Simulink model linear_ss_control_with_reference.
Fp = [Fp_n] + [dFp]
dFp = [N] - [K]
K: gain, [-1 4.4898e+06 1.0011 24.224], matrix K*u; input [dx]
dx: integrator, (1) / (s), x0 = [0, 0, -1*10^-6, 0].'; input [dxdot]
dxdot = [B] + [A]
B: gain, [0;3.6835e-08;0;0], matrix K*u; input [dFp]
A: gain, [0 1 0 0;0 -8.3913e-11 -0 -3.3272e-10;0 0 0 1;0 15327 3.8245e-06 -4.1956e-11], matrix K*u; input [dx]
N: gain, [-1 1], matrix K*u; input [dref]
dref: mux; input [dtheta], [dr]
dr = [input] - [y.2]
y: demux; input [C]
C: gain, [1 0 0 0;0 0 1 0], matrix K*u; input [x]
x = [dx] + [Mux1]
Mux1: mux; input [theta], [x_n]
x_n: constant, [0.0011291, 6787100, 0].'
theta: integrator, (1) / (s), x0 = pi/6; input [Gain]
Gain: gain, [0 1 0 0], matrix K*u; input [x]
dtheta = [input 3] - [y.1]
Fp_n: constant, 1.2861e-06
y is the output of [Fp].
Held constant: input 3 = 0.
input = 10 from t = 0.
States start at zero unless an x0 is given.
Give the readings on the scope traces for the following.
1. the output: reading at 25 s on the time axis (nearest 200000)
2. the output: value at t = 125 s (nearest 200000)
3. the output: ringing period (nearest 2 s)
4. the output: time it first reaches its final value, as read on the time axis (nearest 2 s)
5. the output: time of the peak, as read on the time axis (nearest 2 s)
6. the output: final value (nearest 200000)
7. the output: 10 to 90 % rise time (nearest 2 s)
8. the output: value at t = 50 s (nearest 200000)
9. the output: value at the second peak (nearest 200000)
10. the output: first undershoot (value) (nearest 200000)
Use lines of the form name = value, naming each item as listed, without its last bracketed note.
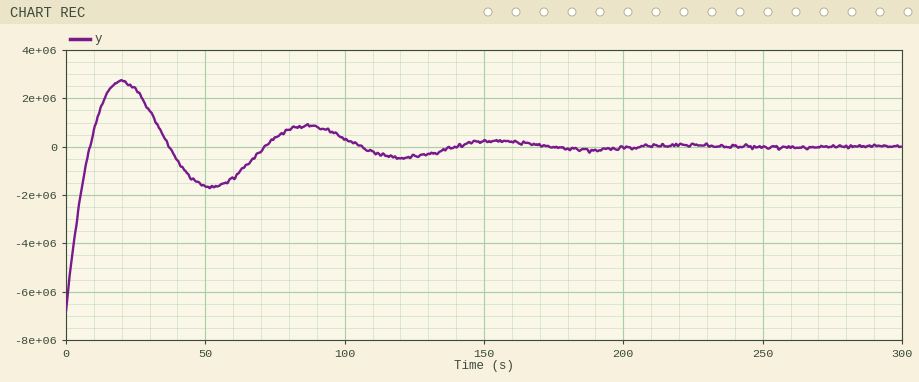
the output: reading at 25 s on the time axis = 2400000
the output: value at t = 125 s = -400000
the output: ringing period = 66 s
the output: time it first reaches its final value, as read on the time axis = 8 s
the output: time of the peak, as read on the time axis = 20 s
the output: final value = 0
the output: 10 to 90 % rise time = 6 s
the output: value at t = 50 s = -1600000
the output: value at the second peak = 800000
the output: first undershoot (value) = -1600000
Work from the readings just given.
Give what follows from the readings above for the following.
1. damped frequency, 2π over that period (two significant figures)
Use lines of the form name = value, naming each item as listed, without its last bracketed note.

damped frequency, 2π over that period = 0.095 rad/s
